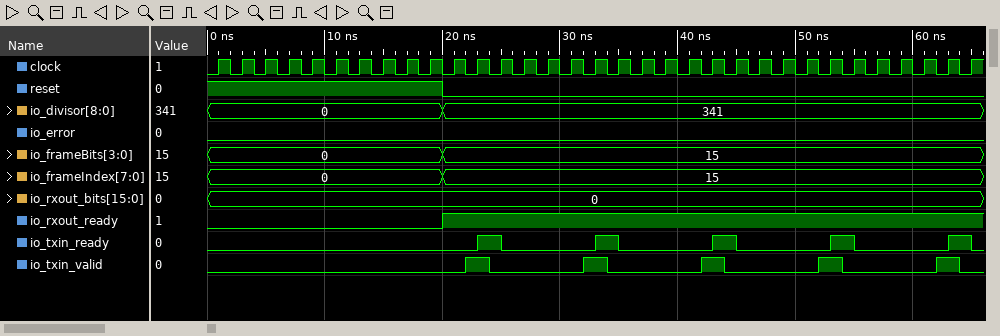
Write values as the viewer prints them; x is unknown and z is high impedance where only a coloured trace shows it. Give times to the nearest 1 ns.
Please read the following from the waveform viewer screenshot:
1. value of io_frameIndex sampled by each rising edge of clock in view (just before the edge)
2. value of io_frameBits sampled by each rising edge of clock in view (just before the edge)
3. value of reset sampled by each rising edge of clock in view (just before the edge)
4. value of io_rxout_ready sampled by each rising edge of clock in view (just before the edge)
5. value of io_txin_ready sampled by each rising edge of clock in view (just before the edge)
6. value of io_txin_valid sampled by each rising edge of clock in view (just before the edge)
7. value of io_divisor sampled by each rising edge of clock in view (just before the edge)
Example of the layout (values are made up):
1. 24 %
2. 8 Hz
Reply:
1. 0, 0, 0, 0, 0, 0, 0, 0, 0, 0, 15, 15, 15, 15, 15, 15, 15, 15, 15, 15, 15, 15, 15, 15, 15, 15, 15, 15, 15, 15, 15, 15, 15
2. 0, 0, 0, 0, 0, 0, 0, 0, 0, 0, 15, 15, 15, 15, 15, 15, 15, 15, 15, 15, 15, 15, 15, 15, 15, 15, 15, 15, 15, 15, 15, 15, 15
3. 1 1 1 1 1 1 1 1 1 1 0 0 0 0 0 0 0 0 0 0 0 0 0 0 0 0 0 0 0 0 0 0 0
4. 0 0 0 0 0 0 0 0 0 0 1 1 1 1 1 1 1 1 1 1 1 1 1 1 1 1 1 1 1 1 1 1 1
5. 0 0 0 0 0 0 0 0 0 0 0 0 1 0 0 0 0 1 0 0 0 0 1 0 0 0 0 1 0 0 0 0 1
6. 0 0 0 0 0 0 0 0 0 0 0 1 0 0 0 0 1 0 0 0 0 1 0 0 0 0 1 0 0 0 0 1 0
7. 0, 0, 0, 0, 0, 0, 0, 0, 0, 0, 341, 341, 341, 341, 341, 341, 341, 341, 341, 341, 341, 341, 341, 341, 341, 341, 341, 341, 341, 341, 341, 341, 341
